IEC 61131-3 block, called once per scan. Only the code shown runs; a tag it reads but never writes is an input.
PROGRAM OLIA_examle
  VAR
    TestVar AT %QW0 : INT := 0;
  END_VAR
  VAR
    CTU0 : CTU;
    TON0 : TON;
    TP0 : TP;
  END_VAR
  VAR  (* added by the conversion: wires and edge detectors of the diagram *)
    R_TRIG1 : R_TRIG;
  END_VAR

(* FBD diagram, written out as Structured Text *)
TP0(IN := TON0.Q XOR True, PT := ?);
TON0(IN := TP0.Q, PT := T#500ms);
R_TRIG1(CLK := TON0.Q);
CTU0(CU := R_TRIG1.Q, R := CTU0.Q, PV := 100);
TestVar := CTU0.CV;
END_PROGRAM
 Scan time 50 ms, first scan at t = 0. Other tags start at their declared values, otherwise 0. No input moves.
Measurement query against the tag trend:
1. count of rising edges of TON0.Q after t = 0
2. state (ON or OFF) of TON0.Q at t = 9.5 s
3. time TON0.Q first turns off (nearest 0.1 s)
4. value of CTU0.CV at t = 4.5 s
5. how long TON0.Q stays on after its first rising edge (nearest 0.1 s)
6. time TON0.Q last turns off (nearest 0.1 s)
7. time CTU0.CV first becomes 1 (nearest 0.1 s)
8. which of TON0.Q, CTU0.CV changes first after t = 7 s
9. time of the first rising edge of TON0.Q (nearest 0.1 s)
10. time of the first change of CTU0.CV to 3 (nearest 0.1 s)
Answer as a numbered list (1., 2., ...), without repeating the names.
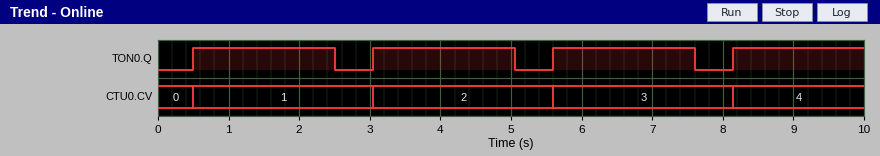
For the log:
1. 4
2. ON
3. 2.5 s
4. 2
5. 2.0 s
6. 7.6 s
7. 0.5 s
8. TON0.Q
9. 0.5 s
10. 5.6 s
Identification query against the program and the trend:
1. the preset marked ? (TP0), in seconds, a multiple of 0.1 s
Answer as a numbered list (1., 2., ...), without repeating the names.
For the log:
1. 2.5 s
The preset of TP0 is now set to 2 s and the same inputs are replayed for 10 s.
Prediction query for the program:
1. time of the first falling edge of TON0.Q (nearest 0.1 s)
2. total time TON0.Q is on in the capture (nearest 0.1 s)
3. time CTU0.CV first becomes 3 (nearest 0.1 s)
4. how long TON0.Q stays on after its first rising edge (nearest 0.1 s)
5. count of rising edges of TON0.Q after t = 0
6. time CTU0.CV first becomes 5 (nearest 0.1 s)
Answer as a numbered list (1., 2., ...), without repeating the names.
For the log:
1. 2.0 s
2. 7.3 s
3. 4.6 s
4. 1.5 s
5. 5
6. 8.7 s
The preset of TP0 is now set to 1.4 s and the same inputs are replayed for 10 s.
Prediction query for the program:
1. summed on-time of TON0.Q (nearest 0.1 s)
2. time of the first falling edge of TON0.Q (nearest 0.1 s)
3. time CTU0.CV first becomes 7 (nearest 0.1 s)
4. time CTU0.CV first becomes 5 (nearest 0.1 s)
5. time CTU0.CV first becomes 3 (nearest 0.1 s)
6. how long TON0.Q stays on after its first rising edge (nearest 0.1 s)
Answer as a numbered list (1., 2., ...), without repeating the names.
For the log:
1. 6.2 s
2. 1.4 s
3. 9.2 s
4. 6.3 s
5. 3.4 s
6. 0.9 s
